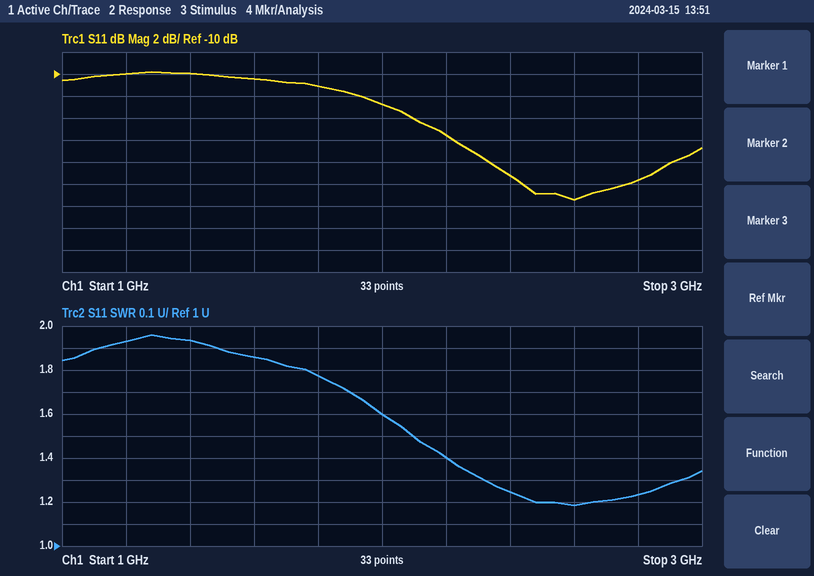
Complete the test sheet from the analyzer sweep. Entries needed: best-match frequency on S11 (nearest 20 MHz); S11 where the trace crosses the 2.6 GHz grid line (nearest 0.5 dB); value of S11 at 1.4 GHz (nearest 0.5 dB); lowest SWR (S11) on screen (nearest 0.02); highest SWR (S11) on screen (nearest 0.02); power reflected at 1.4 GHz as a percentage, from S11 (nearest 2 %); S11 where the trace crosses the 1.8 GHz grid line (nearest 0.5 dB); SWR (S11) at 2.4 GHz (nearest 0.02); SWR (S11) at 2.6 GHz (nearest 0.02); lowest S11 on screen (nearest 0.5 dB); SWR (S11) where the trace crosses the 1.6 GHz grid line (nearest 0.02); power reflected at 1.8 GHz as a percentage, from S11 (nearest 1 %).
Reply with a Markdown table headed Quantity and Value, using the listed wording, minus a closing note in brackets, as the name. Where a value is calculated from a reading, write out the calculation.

| Quantity | Value |
|---|---|
| best-match frequency on S11 | 2.60 GHz |
| S11 where the trace crosses the 2.6 GHz grid line | -21.5 dB |
| value of S11 at 1.4 GHz | -10.0 dB |
| lowest SWR (S11) on screen | 1.18 |
| highest SWR (S11) on screen | 1.96 |
| power reflected at 1.4 GHz as a percentage, from S11 | 10^(-10/10) ≈ 10 % |
| S11 where the trace crosses the 1.8 GHz grid line | -11.0 dB |
| SWR (S11) at 2.4 GHz | 1.24 |
| SWR (S11) at 2.6 GHz | 1.18 |
| lowest S11 on screen | -21.5 dB |
| SWR (S11) where the trace crosses the 1.6 GHz grid line | 1.86 |
| power reflected at 1.8 GHz as a percentage, from S11 | 10^(-11/10) ≈ 8 % |
